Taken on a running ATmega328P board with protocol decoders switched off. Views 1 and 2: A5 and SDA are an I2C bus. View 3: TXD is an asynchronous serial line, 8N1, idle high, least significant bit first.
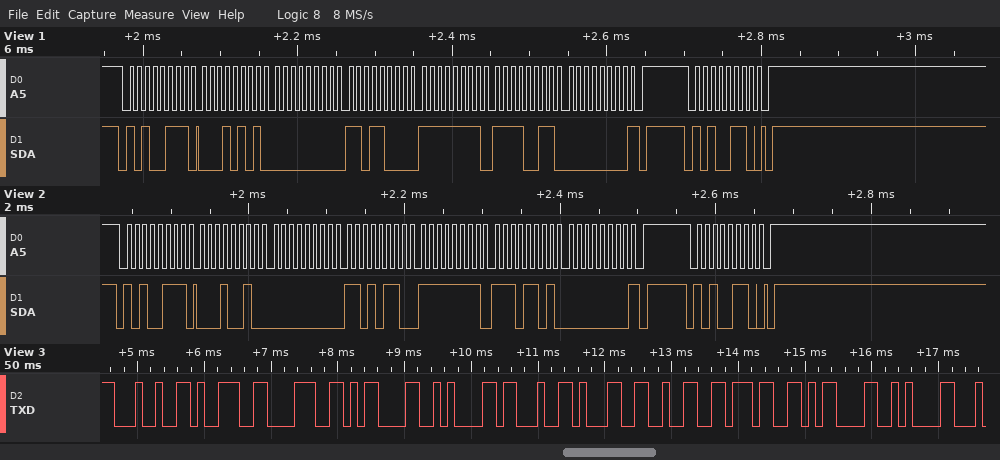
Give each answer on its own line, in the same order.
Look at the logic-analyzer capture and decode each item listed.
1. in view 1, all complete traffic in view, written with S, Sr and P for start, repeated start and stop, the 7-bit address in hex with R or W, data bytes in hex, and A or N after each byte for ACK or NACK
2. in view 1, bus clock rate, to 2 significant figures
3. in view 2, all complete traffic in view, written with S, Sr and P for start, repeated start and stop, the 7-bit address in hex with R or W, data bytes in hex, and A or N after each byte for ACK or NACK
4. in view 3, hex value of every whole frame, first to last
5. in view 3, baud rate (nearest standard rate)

S 53R A 15 A 00 A D8 A FF A F3 A 00 N P S 53W A P
100 kHz
S 53R A 12 A 00 A D6 A FF A ED A 00 N P S 53W A P
24 39 38 0D 0A 23 31 32 37 0D 0A
9600 baud
